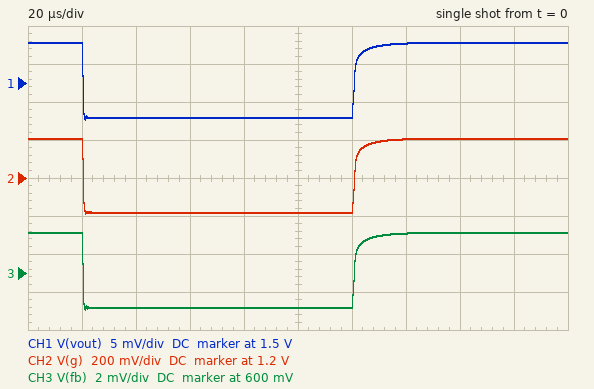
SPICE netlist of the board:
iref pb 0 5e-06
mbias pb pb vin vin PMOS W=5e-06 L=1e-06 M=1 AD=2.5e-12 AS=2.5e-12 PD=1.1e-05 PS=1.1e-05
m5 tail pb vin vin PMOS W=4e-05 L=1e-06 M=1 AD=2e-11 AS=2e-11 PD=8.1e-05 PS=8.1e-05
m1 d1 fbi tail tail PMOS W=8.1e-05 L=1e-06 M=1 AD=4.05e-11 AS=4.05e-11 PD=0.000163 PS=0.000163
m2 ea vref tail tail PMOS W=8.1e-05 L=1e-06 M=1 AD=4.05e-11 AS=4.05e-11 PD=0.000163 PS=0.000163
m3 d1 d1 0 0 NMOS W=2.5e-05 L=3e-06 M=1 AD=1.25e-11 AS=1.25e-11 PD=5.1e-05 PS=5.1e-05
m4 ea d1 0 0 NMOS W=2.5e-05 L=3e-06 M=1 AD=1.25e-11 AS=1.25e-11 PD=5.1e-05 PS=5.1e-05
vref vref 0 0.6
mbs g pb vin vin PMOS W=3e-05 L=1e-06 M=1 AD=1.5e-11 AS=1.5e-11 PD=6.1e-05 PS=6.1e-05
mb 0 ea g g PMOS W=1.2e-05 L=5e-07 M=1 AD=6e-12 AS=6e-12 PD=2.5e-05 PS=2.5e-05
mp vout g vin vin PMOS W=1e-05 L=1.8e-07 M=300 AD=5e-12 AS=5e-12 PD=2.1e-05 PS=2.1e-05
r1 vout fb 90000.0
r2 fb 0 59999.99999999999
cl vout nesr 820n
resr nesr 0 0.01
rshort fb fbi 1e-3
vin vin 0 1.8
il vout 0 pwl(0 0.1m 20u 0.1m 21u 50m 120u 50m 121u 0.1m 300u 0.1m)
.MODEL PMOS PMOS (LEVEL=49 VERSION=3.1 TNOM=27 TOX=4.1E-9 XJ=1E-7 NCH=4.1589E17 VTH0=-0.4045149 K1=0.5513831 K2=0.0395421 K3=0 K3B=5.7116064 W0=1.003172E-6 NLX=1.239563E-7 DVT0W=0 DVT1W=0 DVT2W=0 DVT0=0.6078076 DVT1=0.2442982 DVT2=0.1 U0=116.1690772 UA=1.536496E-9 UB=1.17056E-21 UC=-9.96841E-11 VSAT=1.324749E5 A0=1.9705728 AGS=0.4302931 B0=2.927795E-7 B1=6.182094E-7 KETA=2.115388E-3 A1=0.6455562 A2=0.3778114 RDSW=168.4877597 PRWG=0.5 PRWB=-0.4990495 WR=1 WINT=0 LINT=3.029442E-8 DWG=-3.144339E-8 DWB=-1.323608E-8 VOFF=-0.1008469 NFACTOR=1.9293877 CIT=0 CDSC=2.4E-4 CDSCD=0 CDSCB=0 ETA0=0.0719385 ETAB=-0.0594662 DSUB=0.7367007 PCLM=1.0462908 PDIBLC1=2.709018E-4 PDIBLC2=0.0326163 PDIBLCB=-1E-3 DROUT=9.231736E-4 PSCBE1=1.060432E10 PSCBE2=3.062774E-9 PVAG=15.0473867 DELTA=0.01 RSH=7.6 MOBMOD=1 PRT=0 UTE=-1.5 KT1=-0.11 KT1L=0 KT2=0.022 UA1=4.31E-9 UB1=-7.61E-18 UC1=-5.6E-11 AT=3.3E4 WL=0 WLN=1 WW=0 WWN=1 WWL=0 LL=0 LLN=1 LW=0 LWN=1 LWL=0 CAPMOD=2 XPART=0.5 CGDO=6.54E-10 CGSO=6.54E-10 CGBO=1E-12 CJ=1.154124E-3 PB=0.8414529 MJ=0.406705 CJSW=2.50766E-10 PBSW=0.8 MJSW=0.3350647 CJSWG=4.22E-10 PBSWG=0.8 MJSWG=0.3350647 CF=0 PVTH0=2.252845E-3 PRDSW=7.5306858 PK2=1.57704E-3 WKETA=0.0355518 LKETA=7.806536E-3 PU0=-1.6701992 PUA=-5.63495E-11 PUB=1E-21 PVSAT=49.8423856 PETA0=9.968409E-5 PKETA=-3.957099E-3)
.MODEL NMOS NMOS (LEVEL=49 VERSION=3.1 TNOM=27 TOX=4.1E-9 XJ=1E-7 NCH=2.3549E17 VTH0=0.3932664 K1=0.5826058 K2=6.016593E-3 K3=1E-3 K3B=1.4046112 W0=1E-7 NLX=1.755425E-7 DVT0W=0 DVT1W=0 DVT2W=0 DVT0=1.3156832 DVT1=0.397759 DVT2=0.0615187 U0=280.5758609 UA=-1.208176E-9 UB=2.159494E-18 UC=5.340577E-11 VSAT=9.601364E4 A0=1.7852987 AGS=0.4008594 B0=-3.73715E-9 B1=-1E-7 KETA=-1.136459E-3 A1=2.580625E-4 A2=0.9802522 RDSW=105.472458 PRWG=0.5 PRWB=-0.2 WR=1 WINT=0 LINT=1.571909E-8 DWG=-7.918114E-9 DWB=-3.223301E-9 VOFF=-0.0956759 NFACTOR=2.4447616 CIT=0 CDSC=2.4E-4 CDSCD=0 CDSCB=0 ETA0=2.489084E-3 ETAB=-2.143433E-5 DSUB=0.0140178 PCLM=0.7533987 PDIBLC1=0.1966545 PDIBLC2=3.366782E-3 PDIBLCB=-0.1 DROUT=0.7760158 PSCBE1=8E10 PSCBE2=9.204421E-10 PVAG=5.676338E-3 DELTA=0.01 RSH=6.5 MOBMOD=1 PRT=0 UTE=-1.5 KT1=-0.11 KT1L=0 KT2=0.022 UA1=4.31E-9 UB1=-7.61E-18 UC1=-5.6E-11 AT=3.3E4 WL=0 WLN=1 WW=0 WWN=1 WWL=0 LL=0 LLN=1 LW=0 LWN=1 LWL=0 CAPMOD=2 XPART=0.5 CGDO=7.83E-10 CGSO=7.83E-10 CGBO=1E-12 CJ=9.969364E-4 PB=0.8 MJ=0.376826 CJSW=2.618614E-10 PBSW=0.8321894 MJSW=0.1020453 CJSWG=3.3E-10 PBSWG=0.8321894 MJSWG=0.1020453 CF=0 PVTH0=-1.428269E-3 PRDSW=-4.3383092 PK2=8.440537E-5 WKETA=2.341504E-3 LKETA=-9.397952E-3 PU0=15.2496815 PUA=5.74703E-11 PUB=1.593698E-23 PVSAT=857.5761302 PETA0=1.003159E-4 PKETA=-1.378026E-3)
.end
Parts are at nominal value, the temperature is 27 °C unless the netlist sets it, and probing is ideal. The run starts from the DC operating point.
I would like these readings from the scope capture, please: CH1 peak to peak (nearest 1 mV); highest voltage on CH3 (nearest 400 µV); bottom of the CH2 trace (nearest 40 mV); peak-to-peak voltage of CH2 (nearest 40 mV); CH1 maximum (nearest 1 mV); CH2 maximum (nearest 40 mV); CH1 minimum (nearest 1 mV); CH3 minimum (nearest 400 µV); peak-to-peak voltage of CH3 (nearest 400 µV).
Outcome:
10 mV
602.0 mV
1.00 V
400 mV
1.505 V
1.40 V
1.495 V
598.0 mV
4.0 mV
